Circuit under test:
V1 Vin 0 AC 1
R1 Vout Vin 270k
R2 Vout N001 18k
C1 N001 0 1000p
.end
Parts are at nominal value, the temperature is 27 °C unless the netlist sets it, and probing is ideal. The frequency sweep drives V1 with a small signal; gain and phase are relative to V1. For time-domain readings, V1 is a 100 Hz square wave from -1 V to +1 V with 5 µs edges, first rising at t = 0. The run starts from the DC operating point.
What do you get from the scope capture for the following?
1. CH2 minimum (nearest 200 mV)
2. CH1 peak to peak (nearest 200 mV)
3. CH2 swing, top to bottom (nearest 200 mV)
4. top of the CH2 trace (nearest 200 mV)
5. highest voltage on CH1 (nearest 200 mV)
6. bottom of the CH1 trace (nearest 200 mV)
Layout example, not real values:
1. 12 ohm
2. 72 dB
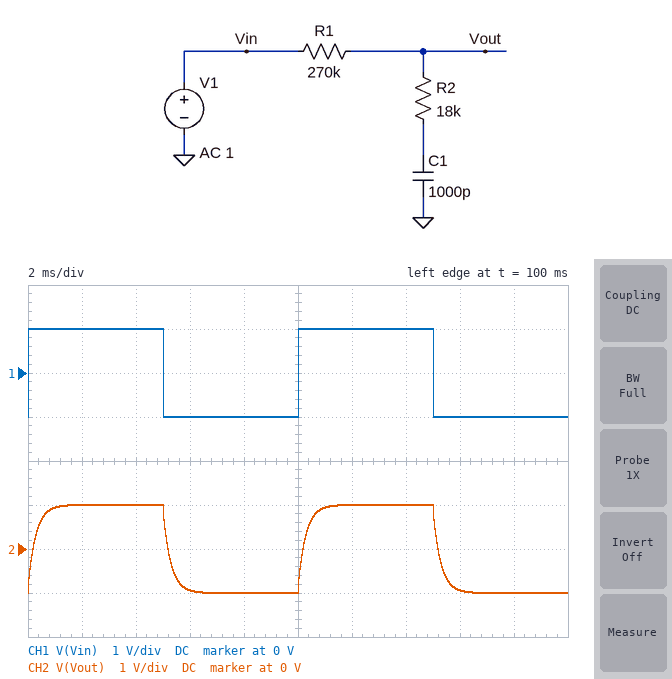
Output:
1. -1.0 V
2. 2.0 V
3. 2.0 V
4. 1.0 V
5. 1.0 V
6. -1.0 V
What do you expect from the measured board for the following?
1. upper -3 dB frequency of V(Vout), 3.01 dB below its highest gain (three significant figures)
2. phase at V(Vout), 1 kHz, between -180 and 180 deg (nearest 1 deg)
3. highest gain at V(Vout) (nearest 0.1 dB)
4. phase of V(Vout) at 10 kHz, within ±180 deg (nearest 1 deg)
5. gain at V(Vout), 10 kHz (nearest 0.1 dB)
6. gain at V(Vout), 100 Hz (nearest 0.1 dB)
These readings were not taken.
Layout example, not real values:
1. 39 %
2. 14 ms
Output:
1. 555 Hz
2. -55 deg
3. 0 dB
4. -38 deg
5. -21.6 dB
6. -0.1 dB
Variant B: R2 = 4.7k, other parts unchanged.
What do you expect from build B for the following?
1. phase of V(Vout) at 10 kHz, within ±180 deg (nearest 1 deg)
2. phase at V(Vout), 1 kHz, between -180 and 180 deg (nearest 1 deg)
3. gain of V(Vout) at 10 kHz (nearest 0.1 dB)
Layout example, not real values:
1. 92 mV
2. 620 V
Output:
1. -70 deg
2. -58 deg
3. -24.4 dB
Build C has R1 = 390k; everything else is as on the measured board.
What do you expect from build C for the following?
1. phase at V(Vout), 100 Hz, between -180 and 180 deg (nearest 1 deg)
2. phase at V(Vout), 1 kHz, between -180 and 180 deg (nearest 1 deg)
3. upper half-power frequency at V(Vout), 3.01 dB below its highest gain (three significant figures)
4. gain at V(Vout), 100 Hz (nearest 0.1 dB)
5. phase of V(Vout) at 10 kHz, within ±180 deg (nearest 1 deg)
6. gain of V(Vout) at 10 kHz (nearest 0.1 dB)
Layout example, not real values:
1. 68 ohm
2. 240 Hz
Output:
1. -14 deg
2. -62 deg
3. 391 Hz
4. -0.3 dB
5. -39 deg
6. -24.6 dB
